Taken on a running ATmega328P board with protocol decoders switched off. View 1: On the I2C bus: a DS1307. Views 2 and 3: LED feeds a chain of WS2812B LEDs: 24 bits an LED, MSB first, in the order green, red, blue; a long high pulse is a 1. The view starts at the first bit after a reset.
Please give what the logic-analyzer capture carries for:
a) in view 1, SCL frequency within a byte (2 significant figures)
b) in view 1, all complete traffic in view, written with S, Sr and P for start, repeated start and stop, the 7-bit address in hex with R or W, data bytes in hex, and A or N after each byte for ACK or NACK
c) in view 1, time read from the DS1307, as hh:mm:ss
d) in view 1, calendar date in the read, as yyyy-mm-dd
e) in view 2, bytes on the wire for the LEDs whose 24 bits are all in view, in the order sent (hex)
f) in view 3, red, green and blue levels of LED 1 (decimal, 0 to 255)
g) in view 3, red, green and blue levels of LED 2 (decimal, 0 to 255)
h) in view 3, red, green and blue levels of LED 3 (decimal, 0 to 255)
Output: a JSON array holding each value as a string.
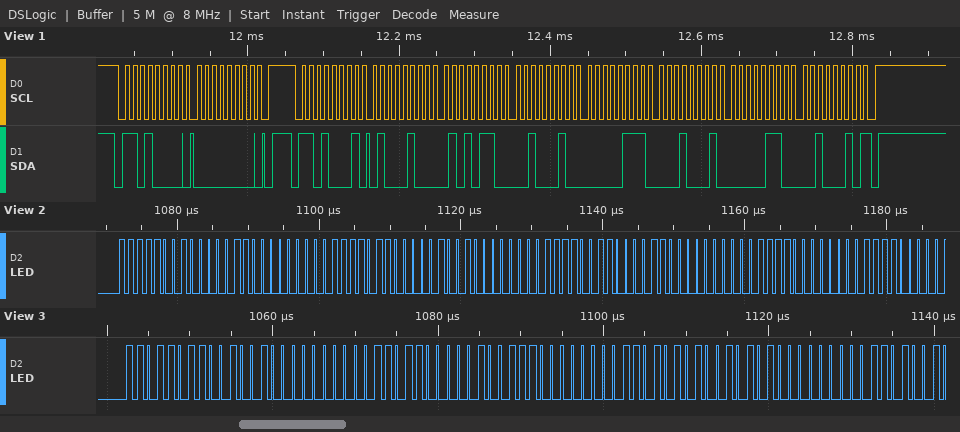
["100 kHz", "S 68W A 00 A P S 68R A 44 A 56 A 22 A 07 A 11 A 06 A 22 N P", "22:56:44", "2022-06-11", "F9 06 00 F6 09 00 F3 0C 00", "36, 219, 0", "39, 216, 0", "42, 213, 0"]
